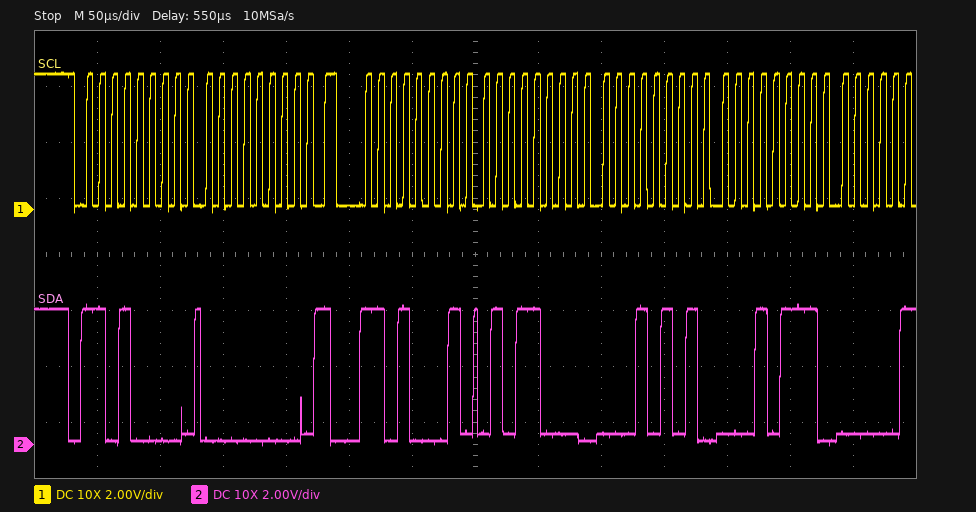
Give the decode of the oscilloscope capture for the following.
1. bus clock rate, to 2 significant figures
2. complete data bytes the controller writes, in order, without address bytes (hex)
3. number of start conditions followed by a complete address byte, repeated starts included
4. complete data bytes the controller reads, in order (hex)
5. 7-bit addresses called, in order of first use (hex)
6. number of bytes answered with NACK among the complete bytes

100 kHz
00
2
58 15 17
0x68
0
